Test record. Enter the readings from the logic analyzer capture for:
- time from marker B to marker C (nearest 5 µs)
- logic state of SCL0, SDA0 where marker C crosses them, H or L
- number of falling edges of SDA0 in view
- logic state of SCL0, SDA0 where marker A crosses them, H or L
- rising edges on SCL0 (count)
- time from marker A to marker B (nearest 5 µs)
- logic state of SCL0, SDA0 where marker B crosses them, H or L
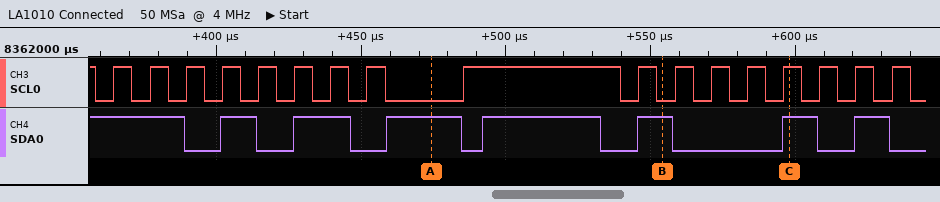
45 µs
SCL0=H, SDA0=H
8
SCL0=L, SDA0=H
17
80 µs
SCL0=L, SDA0=H
